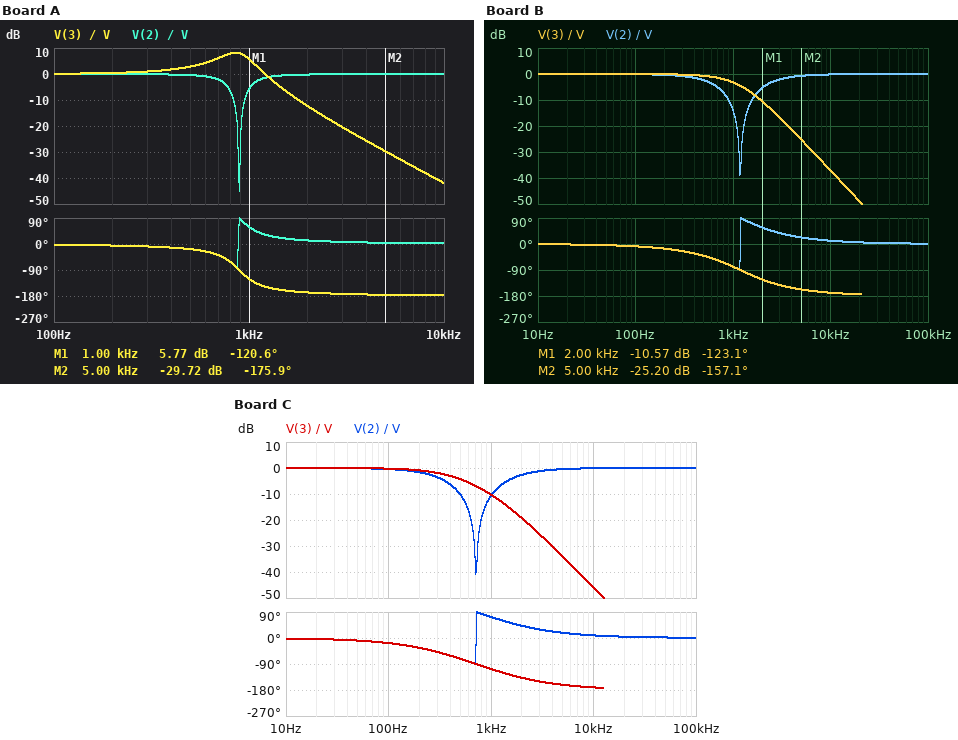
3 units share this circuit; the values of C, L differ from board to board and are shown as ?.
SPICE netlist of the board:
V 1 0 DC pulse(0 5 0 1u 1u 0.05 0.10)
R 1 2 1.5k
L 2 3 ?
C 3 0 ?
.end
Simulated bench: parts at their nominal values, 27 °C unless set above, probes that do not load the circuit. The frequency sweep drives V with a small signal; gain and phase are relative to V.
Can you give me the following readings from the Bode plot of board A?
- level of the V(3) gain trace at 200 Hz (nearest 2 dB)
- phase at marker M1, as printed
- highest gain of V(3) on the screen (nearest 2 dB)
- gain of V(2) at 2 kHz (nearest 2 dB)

0 dB
-120.6 deg
8 dB
0 dB
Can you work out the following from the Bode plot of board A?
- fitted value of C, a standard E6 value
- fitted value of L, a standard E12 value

47 nF
680 mH
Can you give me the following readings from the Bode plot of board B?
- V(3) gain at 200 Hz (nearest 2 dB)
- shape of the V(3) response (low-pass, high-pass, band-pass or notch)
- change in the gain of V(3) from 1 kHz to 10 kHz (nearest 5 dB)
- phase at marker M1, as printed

0 dB
low-pass
-35 dB
-123.1 deg
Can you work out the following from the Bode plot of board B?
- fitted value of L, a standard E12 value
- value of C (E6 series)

120 mH
150 nF
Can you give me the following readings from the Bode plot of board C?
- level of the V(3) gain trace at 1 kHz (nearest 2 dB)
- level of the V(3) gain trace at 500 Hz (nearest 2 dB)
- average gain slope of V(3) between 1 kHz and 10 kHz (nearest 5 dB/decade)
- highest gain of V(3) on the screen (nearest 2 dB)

-10 dB
-4 dB
-35 dB/decade
0 dB
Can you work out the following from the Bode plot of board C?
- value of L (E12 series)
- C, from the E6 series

150 mH
330 nF
